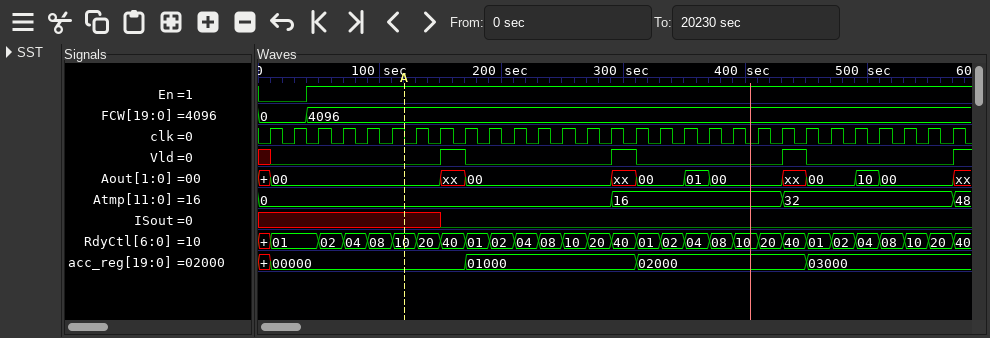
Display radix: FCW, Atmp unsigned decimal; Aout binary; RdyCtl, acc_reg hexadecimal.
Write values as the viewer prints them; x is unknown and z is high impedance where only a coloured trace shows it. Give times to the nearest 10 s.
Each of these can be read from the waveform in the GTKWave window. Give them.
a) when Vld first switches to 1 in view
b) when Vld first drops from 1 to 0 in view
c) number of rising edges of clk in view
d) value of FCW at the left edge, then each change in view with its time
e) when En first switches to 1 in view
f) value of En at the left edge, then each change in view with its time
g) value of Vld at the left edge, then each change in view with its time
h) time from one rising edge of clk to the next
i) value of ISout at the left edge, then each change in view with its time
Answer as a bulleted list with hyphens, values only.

- 150 s
- 170 s
- 29
- 0, 4096 at 40 s
- 40 s
- 0, 1 at 40 s
- x, 0 at 10 s, 1 at 150 s, 0 at 170 s, 1 at 290 s, 0 at 310 s, 1 at 430 s, 0 at 450 s, 1 at 570 s
- 20 s
- x, 0 at 150 s
